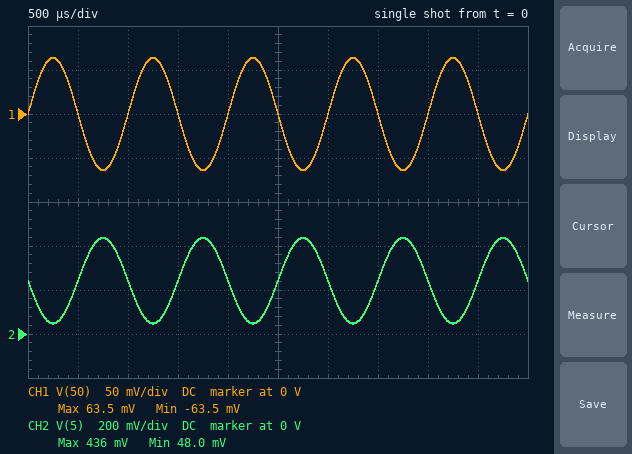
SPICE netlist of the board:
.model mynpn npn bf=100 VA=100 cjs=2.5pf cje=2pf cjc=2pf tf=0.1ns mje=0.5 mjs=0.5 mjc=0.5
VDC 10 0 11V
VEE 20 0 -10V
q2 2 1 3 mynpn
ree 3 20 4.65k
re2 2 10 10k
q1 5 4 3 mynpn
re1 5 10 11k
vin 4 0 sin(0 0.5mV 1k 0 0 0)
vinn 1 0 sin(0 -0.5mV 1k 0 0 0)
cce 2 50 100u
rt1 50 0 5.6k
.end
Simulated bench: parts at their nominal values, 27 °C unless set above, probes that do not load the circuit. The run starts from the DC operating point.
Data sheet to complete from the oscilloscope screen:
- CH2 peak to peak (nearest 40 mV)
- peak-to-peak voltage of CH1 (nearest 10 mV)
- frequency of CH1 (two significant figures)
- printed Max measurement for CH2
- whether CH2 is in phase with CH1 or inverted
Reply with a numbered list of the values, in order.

1. 400 mV
2. 130 mV
3. 1.0 kHz
4. 436 mV
5. inverted
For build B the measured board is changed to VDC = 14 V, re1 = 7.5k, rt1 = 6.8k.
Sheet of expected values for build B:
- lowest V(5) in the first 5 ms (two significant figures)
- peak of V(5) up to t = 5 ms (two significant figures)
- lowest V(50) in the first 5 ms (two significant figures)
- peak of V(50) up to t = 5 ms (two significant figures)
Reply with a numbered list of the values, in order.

1. 6.4 V
2. 6.7 V
3. -73 mV
4. 73 mV
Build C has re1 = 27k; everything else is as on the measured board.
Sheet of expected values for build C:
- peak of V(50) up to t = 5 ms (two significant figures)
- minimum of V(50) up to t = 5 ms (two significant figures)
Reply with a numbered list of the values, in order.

1. 49 mV
2. -37 mV
